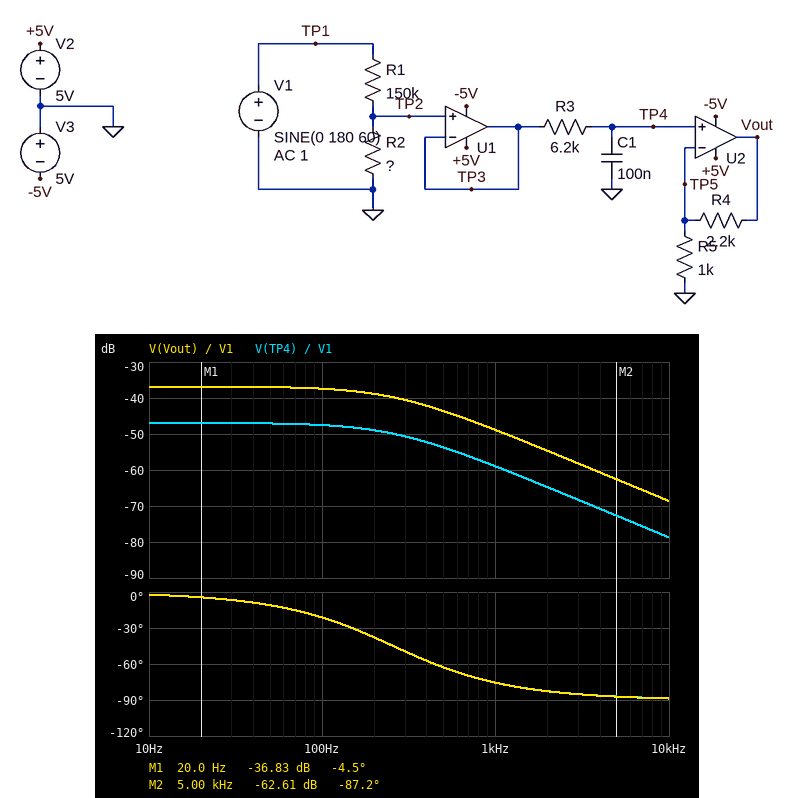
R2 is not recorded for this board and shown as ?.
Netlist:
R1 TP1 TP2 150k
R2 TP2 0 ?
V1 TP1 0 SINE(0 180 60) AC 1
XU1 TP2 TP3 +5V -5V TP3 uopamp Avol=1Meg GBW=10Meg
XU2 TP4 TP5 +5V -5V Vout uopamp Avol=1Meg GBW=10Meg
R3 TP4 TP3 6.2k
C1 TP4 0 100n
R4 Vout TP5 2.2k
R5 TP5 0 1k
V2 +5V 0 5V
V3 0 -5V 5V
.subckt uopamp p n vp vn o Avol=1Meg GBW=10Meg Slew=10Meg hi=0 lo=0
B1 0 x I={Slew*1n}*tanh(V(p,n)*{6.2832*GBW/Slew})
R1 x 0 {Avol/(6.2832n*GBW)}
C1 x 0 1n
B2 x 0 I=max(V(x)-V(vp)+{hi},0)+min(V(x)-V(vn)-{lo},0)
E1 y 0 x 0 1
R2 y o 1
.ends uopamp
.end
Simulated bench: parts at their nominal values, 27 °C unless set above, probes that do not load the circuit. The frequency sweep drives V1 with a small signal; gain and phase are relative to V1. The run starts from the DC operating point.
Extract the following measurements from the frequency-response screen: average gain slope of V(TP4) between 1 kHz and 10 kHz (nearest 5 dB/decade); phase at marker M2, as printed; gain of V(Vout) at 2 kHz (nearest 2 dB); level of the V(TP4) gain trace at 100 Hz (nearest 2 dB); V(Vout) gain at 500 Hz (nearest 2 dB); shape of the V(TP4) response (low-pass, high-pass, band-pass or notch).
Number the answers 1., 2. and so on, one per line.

1. -20 dB/decade
2. -87.2 deg
3. -54 dB
4. -48 dB
5. -44 dB
6. low-pass
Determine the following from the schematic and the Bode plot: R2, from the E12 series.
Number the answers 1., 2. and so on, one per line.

1. 680 Ω
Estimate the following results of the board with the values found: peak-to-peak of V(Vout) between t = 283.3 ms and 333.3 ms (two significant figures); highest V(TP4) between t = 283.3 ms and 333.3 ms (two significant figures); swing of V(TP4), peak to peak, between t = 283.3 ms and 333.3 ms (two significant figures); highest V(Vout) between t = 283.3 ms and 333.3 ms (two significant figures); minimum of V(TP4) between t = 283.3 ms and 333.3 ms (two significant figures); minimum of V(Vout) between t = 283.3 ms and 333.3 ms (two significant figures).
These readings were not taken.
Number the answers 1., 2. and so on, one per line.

1. 5.1 V
2. 790 mV
3. 1.6 V
4. 2.5 V
5. -790 mV
6. -2.5 V
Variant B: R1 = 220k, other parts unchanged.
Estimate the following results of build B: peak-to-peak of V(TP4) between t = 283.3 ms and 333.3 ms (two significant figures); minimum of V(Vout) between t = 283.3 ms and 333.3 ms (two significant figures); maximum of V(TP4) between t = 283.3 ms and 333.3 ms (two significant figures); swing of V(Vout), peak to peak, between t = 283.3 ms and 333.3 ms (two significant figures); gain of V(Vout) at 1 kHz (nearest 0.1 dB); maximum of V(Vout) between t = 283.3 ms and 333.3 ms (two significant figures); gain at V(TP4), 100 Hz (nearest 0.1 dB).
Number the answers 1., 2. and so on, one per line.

1. 1.1 V
2. -1.7 V
3. 540 mV
4. 3.5 V
5. -52.2 dB
6. 1.7 V
7. -50.8 dB
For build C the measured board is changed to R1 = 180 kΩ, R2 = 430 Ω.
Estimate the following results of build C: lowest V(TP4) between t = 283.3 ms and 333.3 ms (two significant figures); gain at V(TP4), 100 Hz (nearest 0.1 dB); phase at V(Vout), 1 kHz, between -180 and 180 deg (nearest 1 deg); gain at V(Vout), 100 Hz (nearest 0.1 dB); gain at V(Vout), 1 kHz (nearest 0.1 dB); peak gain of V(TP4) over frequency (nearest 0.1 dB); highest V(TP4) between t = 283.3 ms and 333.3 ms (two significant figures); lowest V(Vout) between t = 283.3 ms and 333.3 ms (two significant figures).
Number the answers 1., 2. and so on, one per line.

1. -420 mV
2. -53.1 dB
3. -76 deg
4. -43.0 dB
5. -54.4 dB
6. -52.5 dB
7. 420 mV
8. -1.3 V
